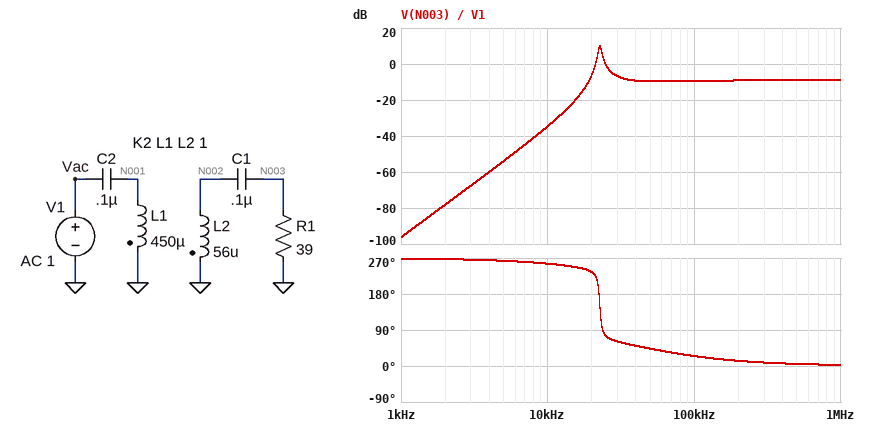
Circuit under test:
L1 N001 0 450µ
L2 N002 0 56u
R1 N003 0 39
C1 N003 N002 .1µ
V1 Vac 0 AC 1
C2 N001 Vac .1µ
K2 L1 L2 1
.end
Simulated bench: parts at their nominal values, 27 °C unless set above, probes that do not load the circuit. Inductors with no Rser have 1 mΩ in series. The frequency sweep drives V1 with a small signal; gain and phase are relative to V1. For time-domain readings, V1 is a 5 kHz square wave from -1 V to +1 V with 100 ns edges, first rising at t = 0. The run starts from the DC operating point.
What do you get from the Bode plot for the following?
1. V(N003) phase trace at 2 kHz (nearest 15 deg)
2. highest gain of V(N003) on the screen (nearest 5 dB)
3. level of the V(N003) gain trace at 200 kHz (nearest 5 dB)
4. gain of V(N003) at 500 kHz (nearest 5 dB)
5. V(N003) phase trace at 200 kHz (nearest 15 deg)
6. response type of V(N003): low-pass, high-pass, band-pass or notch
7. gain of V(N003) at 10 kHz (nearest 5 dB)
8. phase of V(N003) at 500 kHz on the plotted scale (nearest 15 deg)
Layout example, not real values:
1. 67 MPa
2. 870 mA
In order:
1. 270 deg
2. 10 dB
3. -10 dB
4. -10 dB
5. 15 deg
6. high-pass
7. -35 dB
8. 0 deg
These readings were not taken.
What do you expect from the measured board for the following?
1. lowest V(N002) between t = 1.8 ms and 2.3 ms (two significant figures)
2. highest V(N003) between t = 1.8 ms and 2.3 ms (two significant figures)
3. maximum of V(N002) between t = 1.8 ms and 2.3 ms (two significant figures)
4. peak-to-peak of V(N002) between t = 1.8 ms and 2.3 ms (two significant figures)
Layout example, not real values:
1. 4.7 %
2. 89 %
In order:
1. -570 mV
2. 800 mV
3. 570 mV
4. 1.1 V
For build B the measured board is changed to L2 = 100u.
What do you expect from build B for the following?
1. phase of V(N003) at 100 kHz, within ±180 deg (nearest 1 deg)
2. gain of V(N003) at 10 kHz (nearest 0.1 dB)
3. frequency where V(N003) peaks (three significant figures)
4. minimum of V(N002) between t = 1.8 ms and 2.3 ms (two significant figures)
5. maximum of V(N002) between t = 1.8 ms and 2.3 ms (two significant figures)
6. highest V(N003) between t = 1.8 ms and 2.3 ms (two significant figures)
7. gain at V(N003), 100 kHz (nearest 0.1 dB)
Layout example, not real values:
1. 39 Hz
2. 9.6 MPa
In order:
1. 27 deg
2. -31.9 dB
3. 21.9 kHz
4. -710 mV
5. 710 mV
6. 990 mV
7. -7.0 dB
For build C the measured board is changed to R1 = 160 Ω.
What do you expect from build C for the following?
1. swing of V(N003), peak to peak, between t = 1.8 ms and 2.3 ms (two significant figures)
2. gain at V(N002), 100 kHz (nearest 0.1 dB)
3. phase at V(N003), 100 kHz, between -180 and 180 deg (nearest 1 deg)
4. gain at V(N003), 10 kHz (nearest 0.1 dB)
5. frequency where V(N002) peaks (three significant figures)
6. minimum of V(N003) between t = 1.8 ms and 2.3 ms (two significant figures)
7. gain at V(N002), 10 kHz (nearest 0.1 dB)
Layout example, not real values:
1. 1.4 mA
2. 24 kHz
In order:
1. 1.8 V
2. -8.6 dB
3. 6 deg
4. -25.2 dB
5. 23.5 kHz
6. -880 mV
7. -22.2 dB
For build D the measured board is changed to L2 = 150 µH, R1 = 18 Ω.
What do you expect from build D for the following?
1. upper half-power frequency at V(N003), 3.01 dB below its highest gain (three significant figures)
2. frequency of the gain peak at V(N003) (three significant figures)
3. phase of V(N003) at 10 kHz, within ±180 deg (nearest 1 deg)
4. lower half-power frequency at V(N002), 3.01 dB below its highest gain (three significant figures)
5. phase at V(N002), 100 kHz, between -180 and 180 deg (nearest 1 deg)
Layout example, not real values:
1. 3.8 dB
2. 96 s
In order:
1. 21.3 kHz
2. 20.7 kHz
3. -97 deg
4. 20.1 kHz
5. 9 deg
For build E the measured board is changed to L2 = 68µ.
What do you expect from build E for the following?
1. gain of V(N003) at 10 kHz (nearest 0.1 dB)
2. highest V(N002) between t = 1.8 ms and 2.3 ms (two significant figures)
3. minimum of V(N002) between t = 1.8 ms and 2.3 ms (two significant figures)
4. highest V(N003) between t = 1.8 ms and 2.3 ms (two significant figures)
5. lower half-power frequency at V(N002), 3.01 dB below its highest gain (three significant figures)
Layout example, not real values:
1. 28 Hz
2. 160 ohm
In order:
1. -33.7 dB
2. 600 mV
3. -600 mV
4. 860 mV
5. 21.8 kHz
